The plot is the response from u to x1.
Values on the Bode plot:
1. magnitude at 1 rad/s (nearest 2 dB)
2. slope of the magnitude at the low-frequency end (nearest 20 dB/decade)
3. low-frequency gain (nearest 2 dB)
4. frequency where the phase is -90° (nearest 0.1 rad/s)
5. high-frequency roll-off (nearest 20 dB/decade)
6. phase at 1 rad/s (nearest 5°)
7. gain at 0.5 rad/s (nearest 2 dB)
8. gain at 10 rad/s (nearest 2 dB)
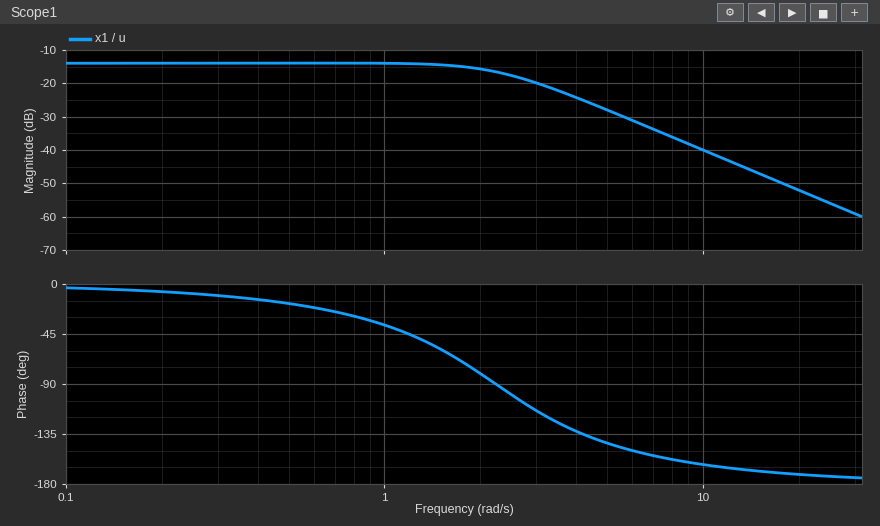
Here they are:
-14 dB
0 dB/decade
-14 dB
2.2 rad/s
-40 dB/decade
-35°
-14 dB
-40 dB
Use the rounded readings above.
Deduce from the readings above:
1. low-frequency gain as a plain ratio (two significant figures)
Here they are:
0.20
